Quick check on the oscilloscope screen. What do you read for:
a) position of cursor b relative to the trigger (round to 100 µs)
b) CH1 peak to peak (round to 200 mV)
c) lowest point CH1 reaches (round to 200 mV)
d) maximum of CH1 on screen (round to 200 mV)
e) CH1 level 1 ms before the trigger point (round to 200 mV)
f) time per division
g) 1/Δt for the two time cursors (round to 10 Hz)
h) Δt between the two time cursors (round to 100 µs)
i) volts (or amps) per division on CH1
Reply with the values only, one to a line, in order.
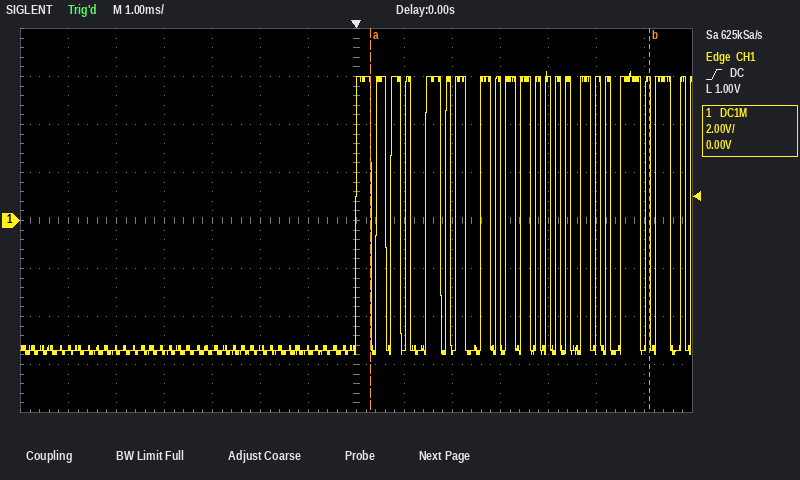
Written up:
+6.1 ms
11.8 V
-5.6 V
6.2 V
-5.4 V
1 ms
170 Hz
5.8 ms
2 V
